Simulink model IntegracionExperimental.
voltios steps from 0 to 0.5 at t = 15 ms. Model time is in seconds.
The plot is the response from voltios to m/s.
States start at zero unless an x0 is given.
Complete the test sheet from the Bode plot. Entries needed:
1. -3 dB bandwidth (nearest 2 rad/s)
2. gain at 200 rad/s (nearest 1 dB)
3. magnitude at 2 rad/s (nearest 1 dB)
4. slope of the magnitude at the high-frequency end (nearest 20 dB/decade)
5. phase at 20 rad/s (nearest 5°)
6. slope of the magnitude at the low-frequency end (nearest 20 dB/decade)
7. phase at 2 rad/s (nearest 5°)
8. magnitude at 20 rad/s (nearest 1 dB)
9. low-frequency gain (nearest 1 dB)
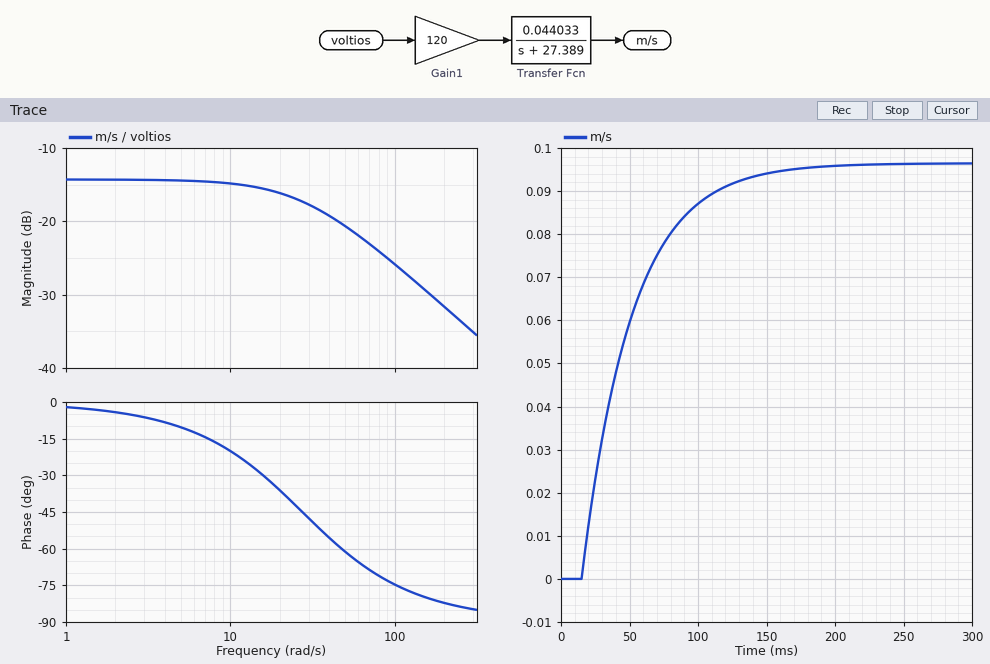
28 rad/s
-32 dB
-14 dB
-20 dB/decade
-35°
0 dB/decade
-5°
-16 dB
-14 dB
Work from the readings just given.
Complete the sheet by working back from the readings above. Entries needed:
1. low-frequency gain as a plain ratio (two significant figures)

0.20
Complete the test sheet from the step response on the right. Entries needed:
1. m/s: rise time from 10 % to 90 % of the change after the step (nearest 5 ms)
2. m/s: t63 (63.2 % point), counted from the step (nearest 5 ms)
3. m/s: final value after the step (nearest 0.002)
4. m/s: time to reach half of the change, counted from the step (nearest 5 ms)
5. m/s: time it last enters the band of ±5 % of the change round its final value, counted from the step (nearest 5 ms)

80 ms
35 ms
0.096
25 ms
110 ms
